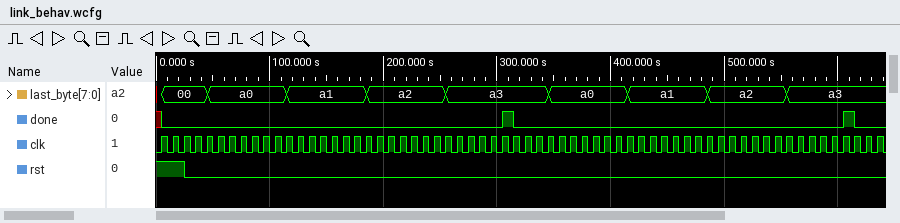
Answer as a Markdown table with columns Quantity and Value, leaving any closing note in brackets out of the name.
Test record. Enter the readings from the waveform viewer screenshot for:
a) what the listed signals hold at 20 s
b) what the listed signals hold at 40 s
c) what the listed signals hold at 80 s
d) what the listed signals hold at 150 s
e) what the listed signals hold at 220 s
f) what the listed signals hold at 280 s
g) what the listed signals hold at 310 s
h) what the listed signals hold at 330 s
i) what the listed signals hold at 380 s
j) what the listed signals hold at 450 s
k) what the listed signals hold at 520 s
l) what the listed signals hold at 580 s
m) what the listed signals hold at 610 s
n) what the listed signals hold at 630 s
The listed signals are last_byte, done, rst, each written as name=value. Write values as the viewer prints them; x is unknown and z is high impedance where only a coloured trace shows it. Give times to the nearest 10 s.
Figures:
| Quantity | Value |
|---|---|
| what the listed signals hold at 20 s | last_byte=00, done=0, rst=1 |
| what the listed signals hold at 40 s | last_byte=00, done=0, rst=0 |
| what the listed signals hold at 80 s | last_byte=a0, done=0, rst=0 |
| what the listed signals hold at 150 s | last_byte=a1, done=0, rst=0 |
| what the listed signals hold at 220 s | last_byte=a2, done=0, rst=0 |
| what the listed signals hold at 280 s | last_byte=a3, done=0, rst=0 |
| what the listed signals hold at 310 s | last_byte=a3, done=1, rst=0 |
| what the listed signals hold at 330 s | last_byte=a3, done=0, rst=0 |
| what the listed signals hold at 380 s | last_byte=a0, done=0, rst=0 |
| what the listed signals hold at 450 s | last_byte=a1, done=0, rst=0 |
| what the listed signals hold at 520 s | last_byte=a2, done=0, rst=0 |
| what the listed signals hold at 580 s | last_byte=a3, done=0, rst=0 |
| what the listed signals hold at 610 s | last_byte=a3, done=1, rst=0 |
| what the listed signals hold at 630 s | last_byte=a3, done=0, rst=0 |
